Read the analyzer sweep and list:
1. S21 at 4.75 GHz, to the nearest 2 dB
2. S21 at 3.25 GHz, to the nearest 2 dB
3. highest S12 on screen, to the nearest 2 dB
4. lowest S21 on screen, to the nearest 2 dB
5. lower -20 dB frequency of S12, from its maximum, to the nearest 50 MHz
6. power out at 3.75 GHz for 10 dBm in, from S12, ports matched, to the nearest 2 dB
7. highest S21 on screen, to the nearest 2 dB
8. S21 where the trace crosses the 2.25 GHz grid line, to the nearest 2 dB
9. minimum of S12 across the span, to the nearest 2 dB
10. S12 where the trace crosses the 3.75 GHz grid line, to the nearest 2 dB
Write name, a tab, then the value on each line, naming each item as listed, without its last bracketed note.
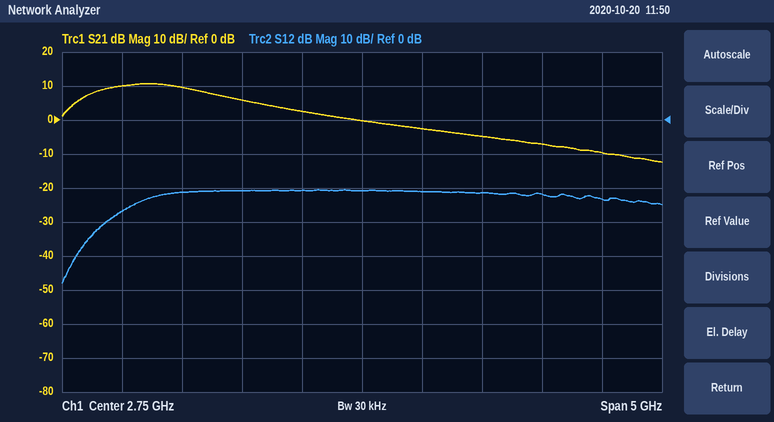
S21 at 4.75 GHz, to the nearest 2 dB	-10 dB
S21 at 3.25 GHz, to the nearest 2 dB	-2 dB
highest S12 on screen, to the nearest 2 dB	-20 dB
lowest S21 on screen, to the nearest 2 dB	-12 dB
lower -20 dB frequency of S12, from its maximum, to the nearest 50 MHz	350 MHz
power out at 3.75 GHz for 10 dBm in, from S12, ports matched, to the nearest 2 dB	-12 dBm
highest S21 on screen, to the nearest 2 dB	10 dB
S21 where the trace crosses the 2.25 GHz grid line, to the nearest 2 dB	2 dB
minimum of S12 across the span, to the nearest 2 dB	-48 dB
S12 where the trace crosses the 3.75 GHz grid line, to the nearest 2 dB	-22 dB
